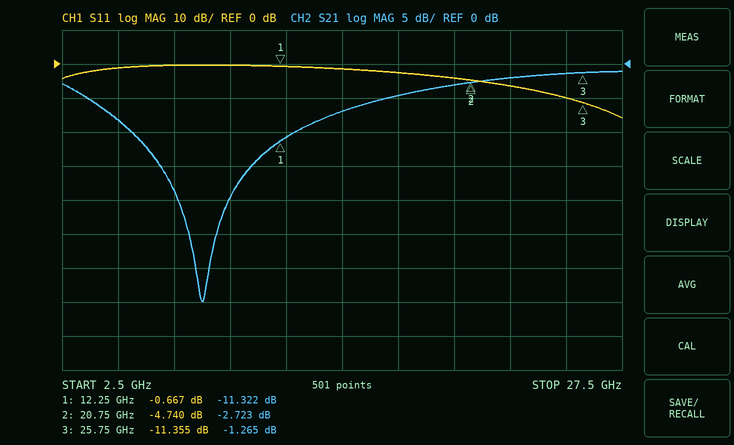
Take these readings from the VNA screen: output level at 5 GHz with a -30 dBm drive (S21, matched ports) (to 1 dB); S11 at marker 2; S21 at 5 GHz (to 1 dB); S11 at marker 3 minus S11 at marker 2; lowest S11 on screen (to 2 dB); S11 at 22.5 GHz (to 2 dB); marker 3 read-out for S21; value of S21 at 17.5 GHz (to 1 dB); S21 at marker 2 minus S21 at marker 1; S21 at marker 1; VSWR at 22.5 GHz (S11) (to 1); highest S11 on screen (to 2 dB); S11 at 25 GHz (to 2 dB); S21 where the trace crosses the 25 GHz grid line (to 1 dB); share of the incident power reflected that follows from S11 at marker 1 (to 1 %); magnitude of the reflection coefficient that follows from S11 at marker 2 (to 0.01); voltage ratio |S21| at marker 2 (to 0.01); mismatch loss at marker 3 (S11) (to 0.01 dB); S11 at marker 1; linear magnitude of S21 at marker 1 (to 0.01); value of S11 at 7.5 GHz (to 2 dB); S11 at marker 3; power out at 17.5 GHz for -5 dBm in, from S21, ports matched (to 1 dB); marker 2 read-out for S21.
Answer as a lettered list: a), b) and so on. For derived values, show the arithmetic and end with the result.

a) -30 dBm + (-8 dB) = -38 dBm
b) -4.740 dB
c) -8 dB
d) -11.355 − (-4.74) = -6.615 dB
e) -16 dB
f) -6 dB
g) -1.265 dB
h) -5 dB
i) -2.723 − (-11.322) = 8.599 dB
j) -11.322 dB
k) |Γ| = 10^(-6/20) = 0.5012; VSWR = (1 + 0.5012)/(1 − 0.5012) ≈ 3
l) 0 dB
m) -10 dB
n) -1 dB
o) 10^(-0.667/10) ≈ 86 %
p) 10^(-4.74/20) ≈ 0.58
q) 10^(-2.723/20) ≈ 0.73
r) −10 log10(1 − 10^(-11.355/10)) ≈ 0.33 dB
s) -0.667 dB
t) 10^(-11.322/20) ≈ 0.27
u) 0 dB
v) -11.355 dB
w) -5 dBm + (-5 dB) = -10 dBm
x) -2.723 dB
